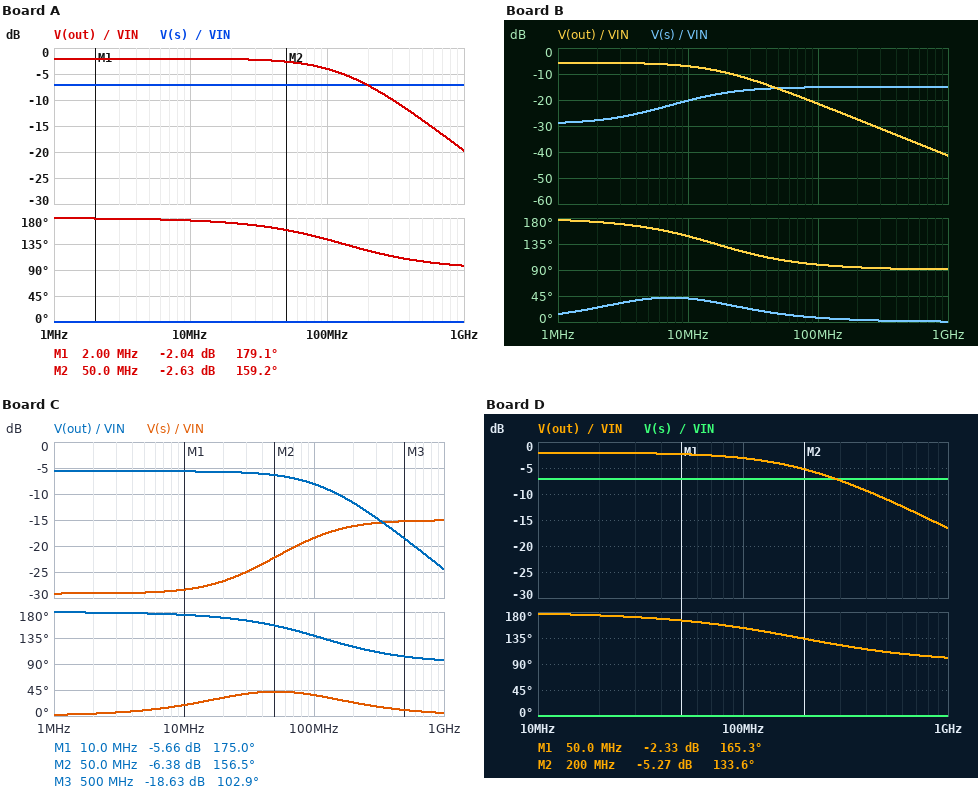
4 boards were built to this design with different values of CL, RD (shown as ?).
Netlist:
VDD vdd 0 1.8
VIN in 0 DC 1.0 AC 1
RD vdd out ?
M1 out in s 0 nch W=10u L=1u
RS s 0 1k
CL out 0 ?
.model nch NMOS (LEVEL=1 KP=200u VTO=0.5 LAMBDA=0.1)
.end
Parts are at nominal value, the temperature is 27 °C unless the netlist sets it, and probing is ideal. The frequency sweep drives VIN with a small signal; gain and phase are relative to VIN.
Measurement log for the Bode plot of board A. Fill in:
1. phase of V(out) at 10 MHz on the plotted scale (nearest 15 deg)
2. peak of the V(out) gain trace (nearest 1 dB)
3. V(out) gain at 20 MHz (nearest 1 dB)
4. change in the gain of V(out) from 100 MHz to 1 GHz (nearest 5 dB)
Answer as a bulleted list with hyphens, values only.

- 180 deg
- -2 dB
- -2 dB
- -15 dB
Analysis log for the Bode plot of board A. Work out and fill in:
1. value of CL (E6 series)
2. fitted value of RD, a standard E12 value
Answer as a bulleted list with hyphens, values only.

- 680 fF
- 1.8 kΩ
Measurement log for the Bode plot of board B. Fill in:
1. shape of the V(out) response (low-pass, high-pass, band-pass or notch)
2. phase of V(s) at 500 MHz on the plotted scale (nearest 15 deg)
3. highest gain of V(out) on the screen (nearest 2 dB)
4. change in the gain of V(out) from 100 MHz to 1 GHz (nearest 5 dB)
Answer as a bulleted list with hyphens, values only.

- low-pass
- 0 deg
- -6 dB
- -20 dB
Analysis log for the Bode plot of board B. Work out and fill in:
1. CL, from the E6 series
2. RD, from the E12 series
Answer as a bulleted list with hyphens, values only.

- 3.3 pF
- 15 kΩ
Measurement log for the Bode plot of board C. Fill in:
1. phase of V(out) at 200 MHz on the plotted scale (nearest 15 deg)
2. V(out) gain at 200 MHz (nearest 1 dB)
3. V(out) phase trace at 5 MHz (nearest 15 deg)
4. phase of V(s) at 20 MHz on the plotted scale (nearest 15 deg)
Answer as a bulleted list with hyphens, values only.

- 120 deg
- -12 dB
- 180 deg
- 30 deg
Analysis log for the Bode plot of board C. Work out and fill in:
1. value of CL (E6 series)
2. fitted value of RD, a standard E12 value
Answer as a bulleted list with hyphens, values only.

- 470 fF
- 15 kΩ
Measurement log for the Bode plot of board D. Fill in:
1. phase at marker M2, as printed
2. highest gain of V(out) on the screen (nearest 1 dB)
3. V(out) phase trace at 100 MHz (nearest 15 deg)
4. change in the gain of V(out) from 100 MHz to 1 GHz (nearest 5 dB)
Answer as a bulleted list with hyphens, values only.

- 133.6 deg
- -2 dB
- 150 deg
- -15 dB
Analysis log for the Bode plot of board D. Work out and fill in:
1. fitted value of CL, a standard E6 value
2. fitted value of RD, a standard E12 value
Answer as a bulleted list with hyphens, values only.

- 470 fF
- 1.8 kΩ
